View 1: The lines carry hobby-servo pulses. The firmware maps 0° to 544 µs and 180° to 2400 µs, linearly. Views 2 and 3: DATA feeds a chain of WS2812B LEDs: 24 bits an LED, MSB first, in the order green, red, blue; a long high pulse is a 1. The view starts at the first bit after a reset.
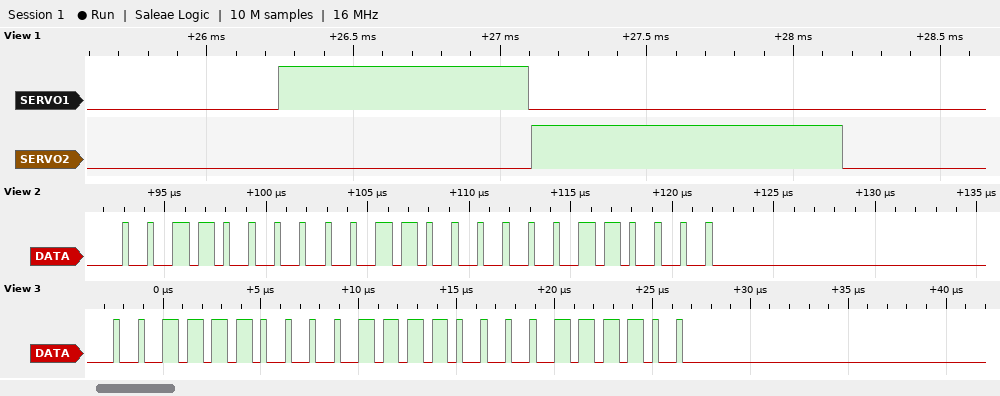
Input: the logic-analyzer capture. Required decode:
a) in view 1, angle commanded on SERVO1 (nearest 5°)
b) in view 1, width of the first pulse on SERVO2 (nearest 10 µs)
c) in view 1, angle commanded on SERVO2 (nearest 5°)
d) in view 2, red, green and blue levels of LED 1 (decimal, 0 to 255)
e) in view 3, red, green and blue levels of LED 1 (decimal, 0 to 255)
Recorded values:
30°
1060 µs
50°
48, 48, 48
60, 60, 60
